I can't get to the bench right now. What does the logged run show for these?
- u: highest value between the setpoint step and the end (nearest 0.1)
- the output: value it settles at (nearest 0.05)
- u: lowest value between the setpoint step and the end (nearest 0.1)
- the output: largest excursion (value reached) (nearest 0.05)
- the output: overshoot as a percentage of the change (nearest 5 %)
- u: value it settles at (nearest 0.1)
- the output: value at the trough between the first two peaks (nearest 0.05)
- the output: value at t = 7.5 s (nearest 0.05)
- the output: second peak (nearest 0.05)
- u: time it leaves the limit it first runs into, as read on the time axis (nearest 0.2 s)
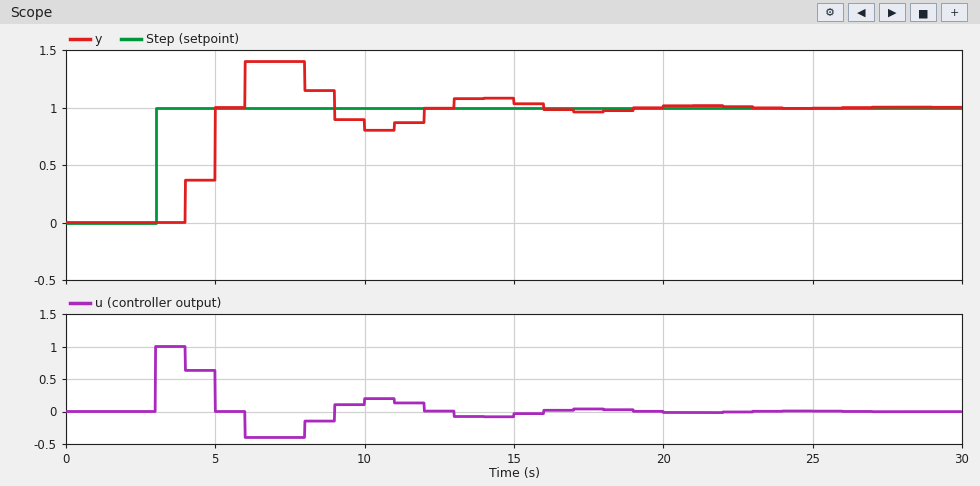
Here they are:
1.0
1.00
-0.4
1.40
40 %
0.0
0.80
1.40
1.10
4.0 s
